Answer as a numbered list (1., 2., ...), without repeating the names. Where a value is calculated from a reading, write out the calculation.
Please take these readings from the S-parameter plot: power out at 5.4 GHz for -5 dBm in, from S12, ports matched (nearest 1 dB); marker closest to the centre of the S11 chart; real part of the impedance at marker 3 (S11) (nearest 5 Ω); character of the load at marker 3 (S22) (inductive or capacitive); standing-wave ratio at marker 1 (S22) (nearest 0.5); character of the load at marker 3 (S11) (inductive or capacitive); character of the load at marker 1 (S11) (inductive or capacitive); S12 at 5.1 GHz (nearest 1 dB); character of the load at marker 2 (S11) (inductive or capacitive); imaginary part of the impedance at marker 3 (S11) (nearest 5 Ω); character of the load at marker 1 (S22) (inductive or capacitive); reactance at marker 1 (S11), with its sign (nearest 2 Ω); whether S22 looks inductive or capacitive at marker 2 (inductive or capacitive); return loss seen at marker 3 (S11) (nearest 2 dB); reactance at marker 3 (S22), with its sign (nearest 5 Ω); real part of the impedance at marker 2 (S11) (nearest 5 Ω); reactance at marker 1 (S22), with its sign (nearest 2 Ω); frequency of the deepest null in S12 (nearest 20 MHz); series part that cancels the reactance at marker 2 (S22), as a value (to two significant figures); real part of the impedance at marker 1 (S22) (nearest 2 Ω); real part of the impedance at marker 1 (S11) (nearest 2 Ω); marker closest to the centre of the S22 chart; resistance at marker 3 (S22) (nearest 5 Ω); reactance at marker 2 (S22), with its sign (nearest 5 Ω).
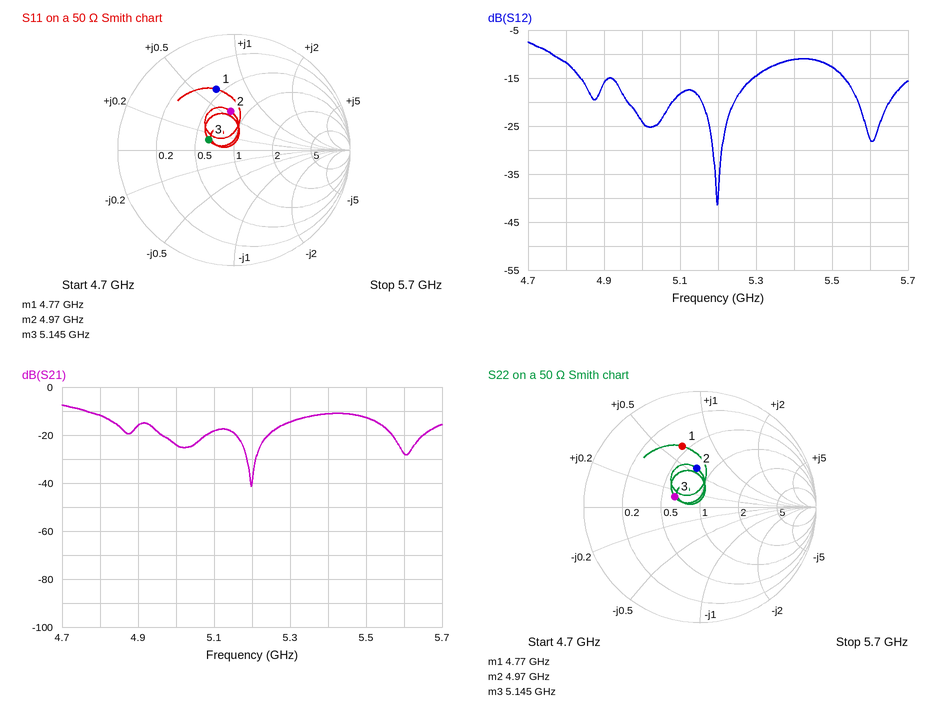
1. -5 dBm + (-11 dB) = -16 dBm
2. marker 3
3. 30 Ω
4. inductive
5. 3.5
6. inductive
7. inductive
8. -18 dB
9. inductive
10. +5 Ω
11. inductive
12. +32 Ω
13. inductive
14. 12 dB
15. +5 Ω
16. 40 Ω
17. +32 Ω
18. 5.20 GHz
19. C = 1/(2π × 4.97 GHz × 30 Ω) ≈ 1.1 pF
20. 22 Ω
21. 22 Ω
22. marker 3
23. 30 Ω
24. +30 Ω
